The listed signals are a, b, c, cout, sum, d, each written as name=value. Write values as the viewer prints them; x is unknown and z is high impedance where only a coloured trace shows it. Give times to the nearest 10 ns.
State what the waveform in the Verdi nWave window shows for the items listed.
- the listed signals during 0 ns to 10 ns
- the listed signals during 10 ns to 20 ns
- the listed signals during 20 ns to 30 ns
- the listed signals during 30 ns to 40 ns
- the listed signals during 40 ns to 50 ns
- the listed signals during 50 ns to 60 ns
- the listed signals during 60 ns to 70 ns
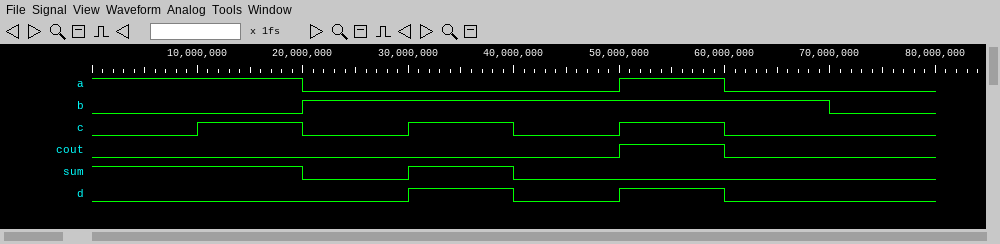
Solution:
a=1, b=0, c=0, cout=0, sum=1, d=0
a=1, b=0, c=1, cout=0, sum=1, d=0
a=0, b=1, c=0, cout=0, sum=0, d=0
a=0, b=1, c=1, cout=0, sum=1, d=1
a=0, b=1, c=0, cout=0, sum=0, d=0
a=1, b=1, c=1, cout=1, sum=0, d=1
a=0, b=1, c=0, cout=0, sum=0, d=0
